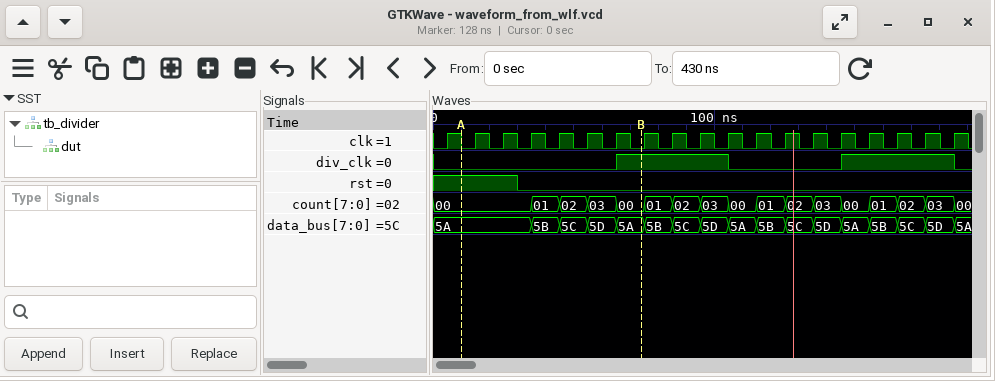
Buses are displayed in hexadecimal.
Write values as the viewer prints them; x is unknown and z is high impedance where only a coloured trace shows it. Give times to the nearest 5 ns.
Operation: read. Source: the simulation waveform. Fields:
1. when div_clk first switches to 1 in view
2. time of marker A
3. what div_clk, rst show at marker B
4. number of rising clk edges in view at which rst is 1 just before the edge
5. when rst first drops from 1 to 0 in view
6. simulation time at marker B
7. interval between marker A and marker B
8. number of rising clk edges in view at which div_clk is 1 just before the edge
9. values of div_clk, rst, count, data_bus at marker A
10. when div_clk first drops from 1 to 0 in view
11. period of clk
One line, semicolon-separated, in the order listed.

65 ns; 10 ns; div_clk=1, rst=0; 3; 30 ns; 75 ns; 65 ns; 8; div_clk=0, rst=1, count=00, data_bus=5A; 105 ns; 10 ns
